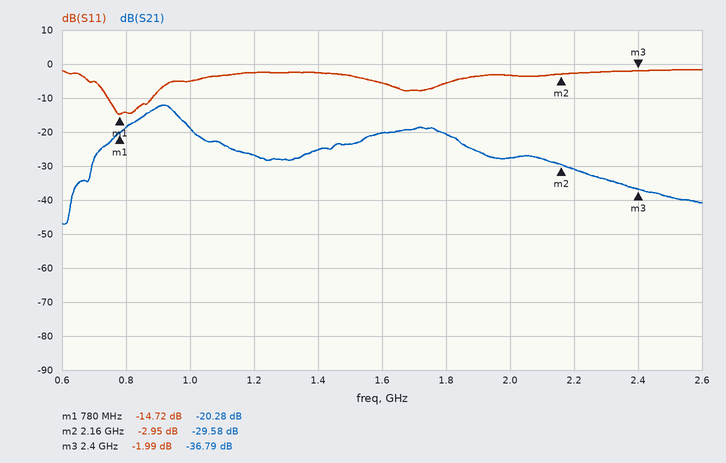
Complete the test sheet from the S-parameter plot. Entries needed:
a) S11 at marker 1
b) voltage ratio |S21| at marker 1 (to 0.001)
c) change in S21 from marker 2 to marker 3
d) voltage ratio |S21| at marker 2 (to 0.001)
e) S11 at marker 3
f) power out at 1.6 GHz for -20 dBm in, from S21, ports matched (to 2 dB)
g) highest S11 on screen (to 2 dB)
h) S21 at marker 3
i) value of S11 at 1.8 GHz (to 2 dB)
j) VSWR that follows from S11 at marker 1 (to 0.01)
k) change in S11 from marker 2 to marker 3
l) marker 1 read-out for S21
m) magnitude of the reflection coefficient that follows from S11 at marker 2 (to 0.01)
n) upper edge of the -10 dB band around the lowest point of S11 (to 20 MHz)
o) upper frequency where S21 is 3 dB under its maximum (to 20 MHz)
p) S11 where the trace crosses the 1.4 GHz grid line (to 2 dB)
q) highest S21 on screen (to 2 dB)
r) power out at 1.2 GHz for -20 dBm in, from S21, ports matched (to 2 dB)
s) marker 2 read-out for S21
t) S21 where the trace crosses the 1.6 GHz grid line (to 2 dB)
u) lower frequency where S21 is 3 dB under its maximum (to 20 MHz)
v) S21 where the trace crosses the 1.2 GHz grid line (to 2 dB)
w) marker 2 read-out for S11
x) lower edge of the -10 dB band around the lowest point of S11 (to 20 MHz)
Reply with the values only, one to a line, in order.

-14.72 dB
0.097
-7.21 dB
0.033
-1.99 dB
-40 dBm
-2 dB
-36.79 dB
-6 dB
1.45
0.96 dB
-20.28 dB
0.71
880 MHz
960 MHz
-2 dB
-12 dB
-46 dBm
-29.58 dB
-20 dB
860 MHz
-26 dB
-2.95 dB
740 MHz
